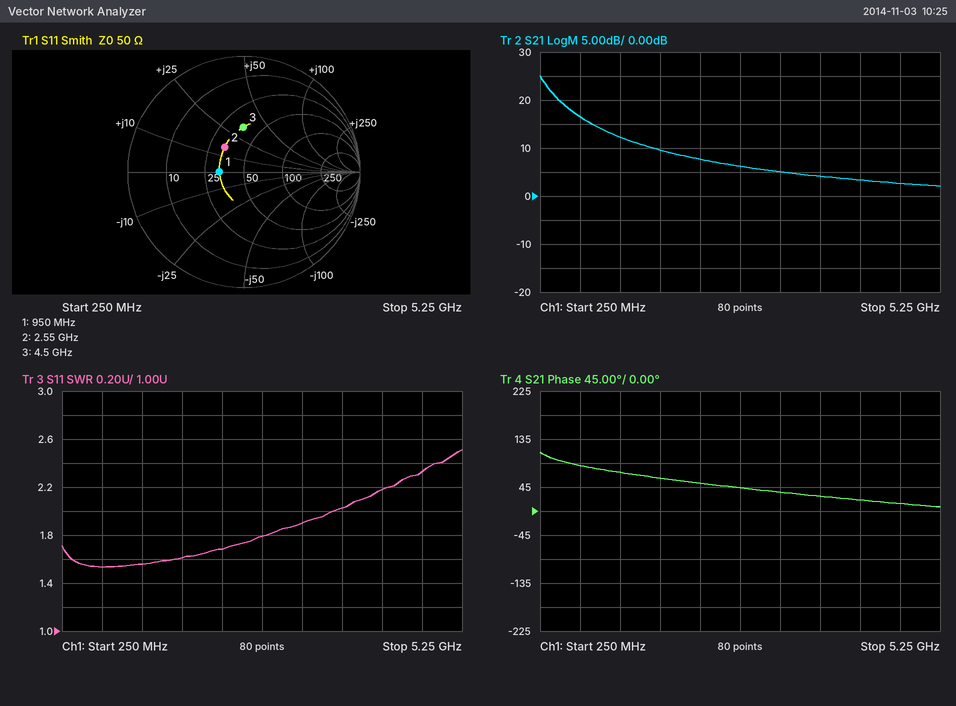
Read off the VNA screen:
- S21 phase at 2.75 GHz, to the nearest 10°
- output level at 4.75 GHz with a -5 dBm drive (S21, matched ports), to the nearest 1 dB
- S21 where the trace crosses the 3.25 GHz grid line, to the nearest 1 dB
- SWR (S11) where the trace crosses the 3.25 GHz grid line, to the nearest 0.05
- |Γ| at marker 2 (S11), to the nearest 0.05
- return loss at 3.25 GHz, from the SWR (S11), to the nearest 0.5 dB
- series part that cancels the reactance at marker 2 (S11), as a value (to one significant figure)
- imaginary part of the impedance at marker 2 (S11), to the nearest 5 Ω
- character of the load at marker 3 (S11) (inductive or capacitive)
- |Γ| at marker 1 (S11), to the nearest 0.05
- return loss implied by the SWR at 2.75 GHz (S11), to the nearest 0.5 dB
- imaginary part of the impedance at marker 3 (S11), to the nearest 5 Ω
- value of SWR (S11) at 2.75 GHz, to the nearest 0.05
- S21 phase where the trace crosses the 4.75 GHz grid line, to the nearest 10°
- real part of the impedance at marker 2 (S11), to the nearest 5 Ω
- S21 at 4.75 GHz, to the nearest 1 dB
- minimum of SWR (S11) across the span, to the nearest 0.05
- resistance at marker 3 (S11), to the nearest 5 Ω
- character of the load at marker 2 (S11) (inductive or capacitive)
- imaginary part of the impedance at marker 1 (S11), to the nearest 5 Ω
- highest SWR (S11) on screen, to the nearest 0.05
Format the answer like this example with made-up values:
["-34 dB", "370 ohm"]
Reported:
["40°", "-2 dBm", "5 dB", "1.90", "0.25", "10.0 dB", "4 pF", "+15 Ω", "inductive", "0.20", "11.0 dB", "+35 Ω", "1.80", "10°", "35 Ω", "3 dB", "1.55", "35 Ω", "inductive", "0 Ω", "2.50"]
